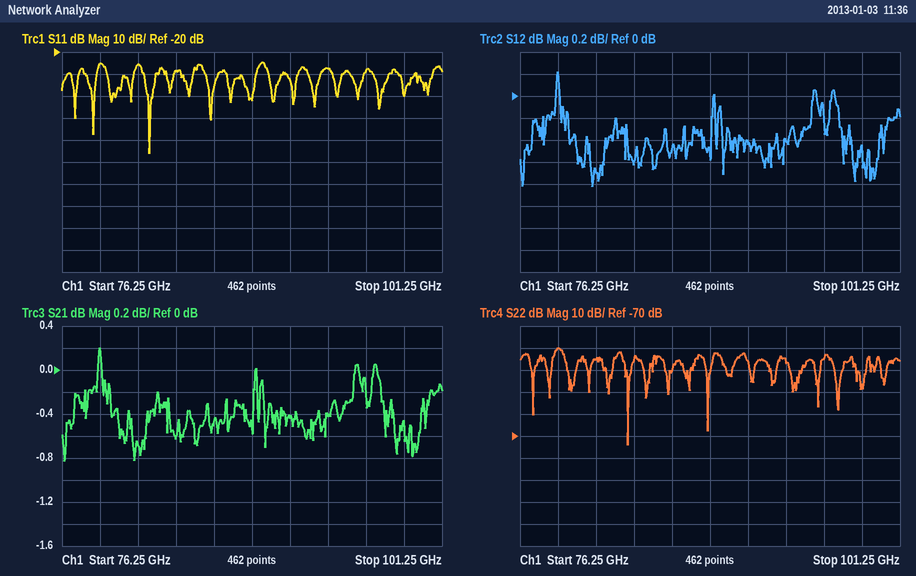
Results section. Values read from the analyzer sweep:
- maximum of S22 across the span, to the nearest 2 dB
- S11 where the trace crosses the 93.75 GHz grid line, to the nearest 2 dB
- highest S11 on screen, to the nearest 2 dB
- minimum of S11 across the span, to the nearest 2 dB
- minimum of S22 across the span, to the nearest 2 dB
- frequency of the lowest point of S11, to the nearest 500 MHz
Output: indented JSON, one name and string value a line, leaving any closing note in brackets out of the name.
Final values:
{
  "maximum of S22 across the span, to the nearest 2 dB": "-30 dB",
  "S11 where the trace crosses the 93.75 GHz grid line, to the nearest 2 dB": "-28 dB",
  "highest S11 on screen, to the nearest 2 dB": "-24 dB",
  "minimum of S11 across the span, to the nearest 2 dB": "-66 dB",
  "minimum of S22 across the span, to the nearest 2 dB": "-74 dB",
  "frequency of the lowest point of S11, to the nearest 500 MHz": "82.0 GHz"
}
